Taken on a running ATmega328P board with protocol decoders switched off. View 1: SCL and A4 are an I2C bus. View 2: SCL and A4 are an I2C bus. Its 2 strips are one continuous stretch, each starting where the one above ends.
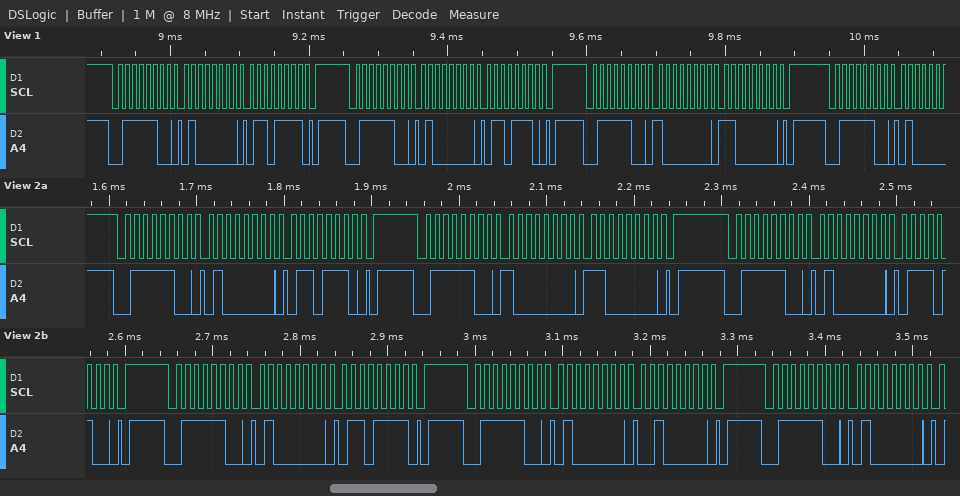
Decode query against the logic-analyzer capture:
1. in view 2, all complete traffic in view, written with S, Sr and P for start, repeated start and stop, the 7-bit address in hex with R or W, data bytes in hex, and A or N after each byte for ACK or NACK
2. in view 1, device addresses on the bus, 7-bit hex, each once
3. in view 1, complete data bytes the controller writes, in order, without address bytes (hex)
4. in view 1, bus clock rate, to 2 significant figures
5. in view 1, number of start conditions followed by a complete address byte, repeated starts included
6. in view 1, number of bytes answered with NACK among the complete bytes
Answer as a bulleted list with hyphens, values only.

- S 3EW A 40 A 6E A P S 3EW A 80 A C0 A P S 3EW A 40 A 74 A P S 3EW A 40 A 6F A P S 3EW A 40 A 20 A P S 3EW A 40 A
- 0x3E
- 40 6F 40 6E 80 C0
- 100 kHz
- 4
- 0
